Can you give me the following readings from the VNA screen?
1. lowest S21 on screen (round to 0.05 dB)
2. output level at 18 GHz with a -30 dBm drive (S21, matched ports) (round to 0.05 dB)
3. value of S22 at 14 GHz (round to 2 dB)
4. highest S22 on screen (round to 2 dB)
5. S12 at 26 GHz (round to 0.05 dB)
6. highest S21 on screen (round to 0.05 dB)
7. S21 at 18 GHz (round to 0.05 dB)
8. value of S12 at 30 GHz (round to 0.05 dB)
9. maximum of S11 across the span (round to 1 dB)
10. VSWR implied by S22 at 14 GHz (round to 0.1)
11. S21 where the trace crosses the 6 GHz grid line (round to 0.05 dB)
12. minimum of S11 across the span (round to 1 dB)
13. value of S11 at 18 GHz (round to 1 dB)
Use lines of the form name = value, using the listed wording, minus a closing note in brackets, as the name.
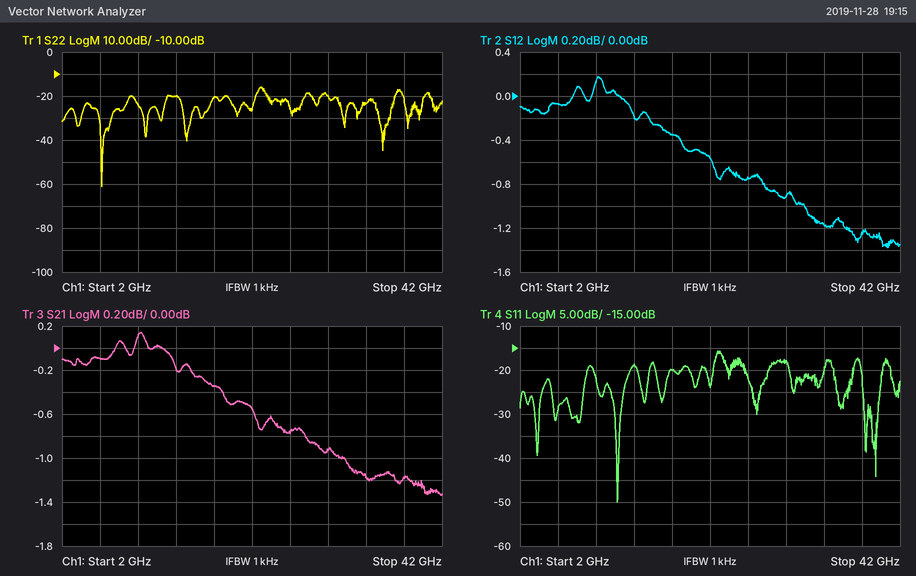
lowest S21 on screen = -1.35 dB
output level at 18 GHz with a -30 dBm drive (S21, matched ports) = -30.35 dBm
value of S22 at 14 GHz = -20 dB
highest S22 on screen = -16 dB
S12 at 26 GHz = -0.75 dB
highest S21 on screen = 0.15 dB
S21 at 18 GHz = -0.35 dB
value of S12 at 30 GHz = -0.90 dB
maximum of S11 across the span = -16 dB
VSWR implied by S22 at 14 GHz = 1.2
S21 where the trace crosses the 6 GHz grid line = -0.10 dB
minimum of S11 across the span = -50 dB
value of S11 at 18 GHz = -20 dB
